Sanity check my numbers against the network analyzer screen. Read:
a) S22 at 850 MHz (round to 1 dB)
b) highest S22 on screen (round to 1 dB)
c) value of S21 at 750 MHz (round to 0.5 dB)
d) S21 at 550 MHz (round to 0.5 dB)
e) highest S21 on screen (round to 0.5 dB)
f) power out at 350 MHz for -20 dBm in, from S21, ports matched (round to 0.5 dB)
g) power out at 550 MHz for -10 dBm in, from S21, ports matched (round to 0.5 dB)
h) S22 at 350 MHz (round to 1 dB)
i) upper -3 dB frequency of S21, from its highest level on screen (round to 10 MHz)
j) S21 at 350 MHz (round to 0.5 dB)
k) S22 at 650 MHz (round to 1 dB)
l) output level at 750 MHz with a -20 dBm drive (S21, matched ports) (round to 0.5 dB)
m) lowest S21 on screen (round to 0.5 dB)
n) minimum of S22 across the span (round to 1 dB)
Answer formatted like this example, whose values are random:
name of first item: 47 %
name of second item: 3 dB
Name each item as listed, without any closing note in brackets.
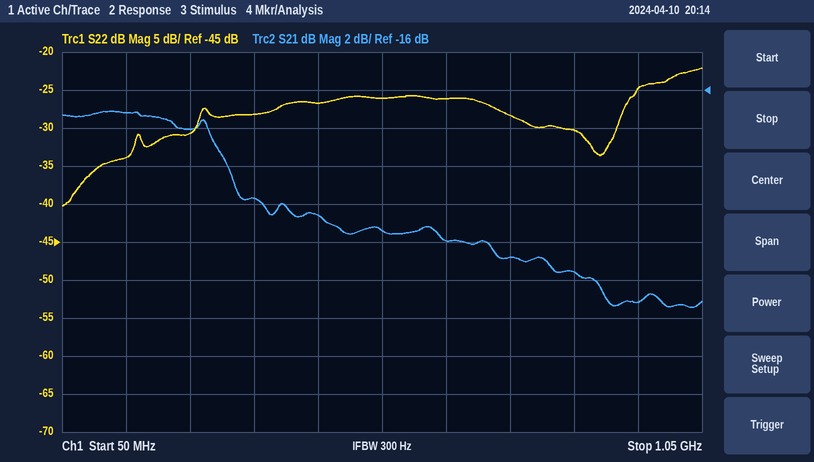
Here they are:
S22 at 850 MHz: -30 dB
highest S22 on screen: -22 dB
value of S21 at 750 MHz: -25.0 dB
S21 at 550 MHz: -23.5 dB
highest S21 on screen: -17.0 dB
power out at 350 MHz for -20 dBm in, from S21, ports matched: -41.5 dBm
power out at 550 MHz for -10 dBm in, from S21, ports matched: -33.5 dBm
S22 at 350 MHz: -28 dB
upper -3 dB frequency of S21, from its highest level on screen: 310 MHz
S21 at 350 MHz: -21.5 dB
S22 at 650 MHz: -26 dB
output level at 750 MHz with a -20 dBm drive (S21, matched ports): -45.0 dBm
lowest S21 on screen: -27.5 dB
minimum of S22 across the span: -40 dB
